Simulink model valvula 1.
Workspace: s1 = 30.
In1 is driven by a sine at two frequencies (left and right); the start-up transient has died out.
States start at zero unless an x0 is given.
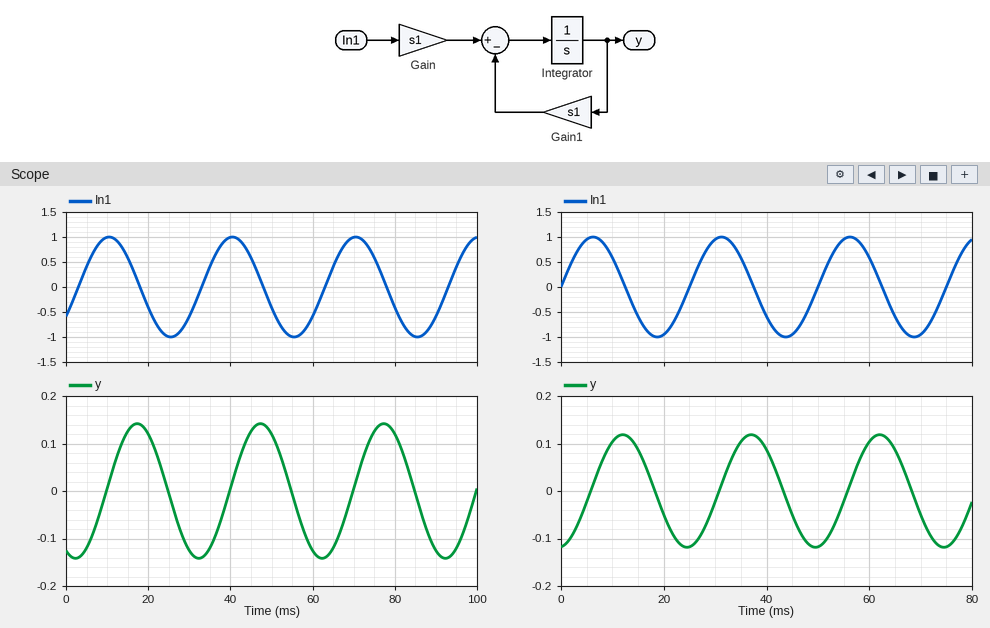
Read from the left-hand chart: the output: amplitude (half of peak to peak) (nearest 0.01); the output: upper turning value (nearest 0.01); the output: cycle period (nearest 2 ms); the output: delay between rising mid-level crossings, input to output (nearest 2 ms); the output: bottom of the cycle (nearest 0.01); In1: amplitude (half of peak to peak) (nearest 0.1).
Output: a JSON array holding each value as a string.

["0.14", "0.14", "30 ms", "6 ms", "-0.14", "1.0"]
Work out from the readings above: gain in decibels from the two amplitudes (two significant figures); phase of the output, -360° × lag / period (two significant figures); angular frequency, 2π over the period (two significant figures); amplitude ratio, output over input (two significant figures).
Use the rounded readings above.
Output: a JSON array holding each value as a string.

["-17 dB", "-72°", "0.21 rad/ms", "0.14"]
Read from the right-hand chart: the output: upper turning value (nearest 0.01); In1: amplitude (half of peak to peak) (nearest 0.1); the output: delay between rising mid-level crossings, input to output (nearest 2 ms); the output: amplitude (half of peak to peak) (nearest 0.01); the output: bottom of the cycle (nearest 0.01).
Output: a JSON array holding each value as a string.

["0.12", "1.0", "6 ms", "0.12", "-0.12"]
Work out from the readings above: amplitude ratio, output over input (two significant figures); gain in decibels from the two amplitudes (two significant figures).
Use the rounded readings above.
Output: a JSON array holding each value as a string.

["0.12", "-18 dB"]
